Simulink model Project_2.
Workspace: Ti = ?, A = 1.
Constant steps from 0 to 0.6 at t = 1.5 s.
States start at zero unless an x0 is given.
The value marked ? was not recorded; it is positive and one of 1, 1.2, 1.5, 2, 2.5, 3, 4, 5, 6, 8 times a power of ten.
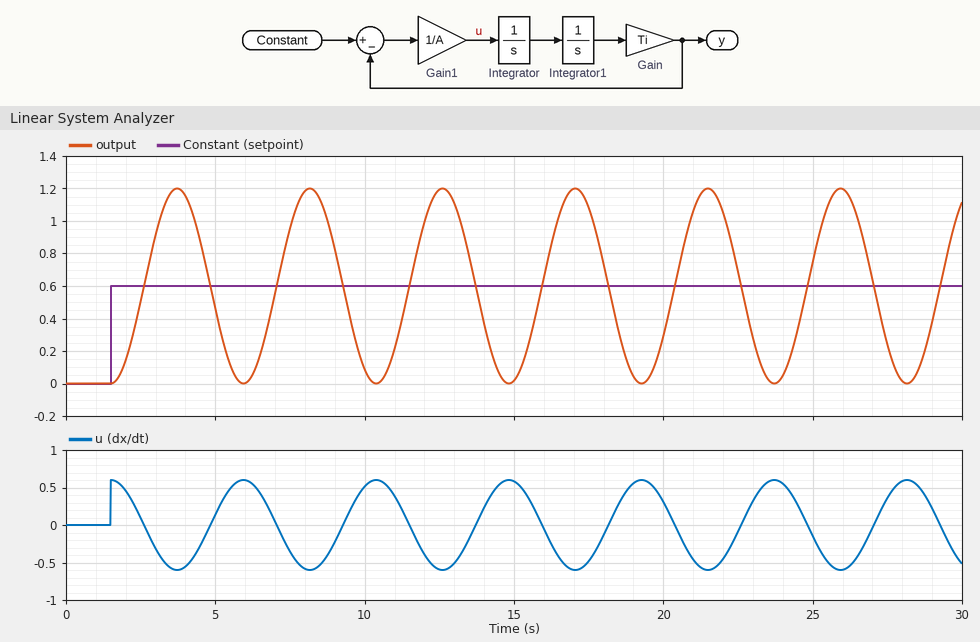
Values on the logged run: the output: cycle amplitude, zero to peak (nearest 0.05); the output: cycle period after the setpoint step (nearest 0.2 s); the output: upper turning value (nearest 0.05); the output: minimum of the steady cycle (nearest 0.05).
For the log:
0.60
4.4 s
1.20
0.00
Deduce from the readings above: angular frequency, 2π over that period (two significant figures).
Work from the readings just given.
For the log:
1.4 rad/s
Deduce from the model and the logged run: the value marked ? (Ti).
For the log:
2
